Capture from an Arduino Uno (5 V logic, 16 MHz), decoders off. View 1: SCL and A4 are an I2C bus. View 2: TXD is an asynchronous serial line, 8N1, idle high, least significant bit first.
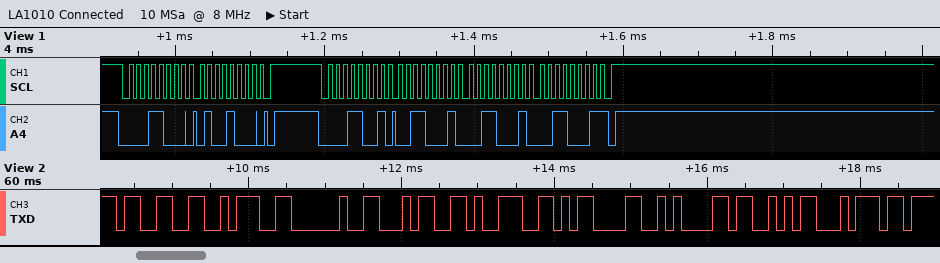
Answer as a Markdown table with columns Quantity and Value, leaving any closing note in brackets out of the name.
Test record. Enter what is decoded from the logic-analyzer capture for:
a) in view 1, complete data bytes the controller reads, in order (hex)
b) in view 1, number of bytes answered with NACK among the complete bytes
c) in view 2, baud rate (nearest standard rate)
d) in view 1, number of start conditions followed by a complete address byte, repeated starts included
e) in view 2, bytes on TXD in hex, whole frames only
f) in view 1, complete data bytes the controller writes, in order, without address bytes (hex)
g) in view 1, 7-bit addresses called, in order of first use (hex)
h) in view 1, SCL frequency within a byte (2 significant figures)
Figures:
| Quantity | Value |
|---|---|
| in view 1, complete data bytes the controller reads, in order | 31 31 31 |
| in view 1, number of bytes answered with NACK among the complete bytes | 1 |
| in view 2, baud rate | 9600 baud |
| in view 1, number of start conditions followed by a complete address byte, repeated starts included | 2 |
| in view 2, bytes on TXD in hex, whole frames only | 33 3A 20 34 39 0D 0A 53 74 |
| in view 1, complete data bytes the controller writes, in order, without address bytes | 48 |
| in view 1, 7-bit addresses called, in order of first use | 0x0C |
| in view 1, SCL frequency within a byte | 100 kHz |
